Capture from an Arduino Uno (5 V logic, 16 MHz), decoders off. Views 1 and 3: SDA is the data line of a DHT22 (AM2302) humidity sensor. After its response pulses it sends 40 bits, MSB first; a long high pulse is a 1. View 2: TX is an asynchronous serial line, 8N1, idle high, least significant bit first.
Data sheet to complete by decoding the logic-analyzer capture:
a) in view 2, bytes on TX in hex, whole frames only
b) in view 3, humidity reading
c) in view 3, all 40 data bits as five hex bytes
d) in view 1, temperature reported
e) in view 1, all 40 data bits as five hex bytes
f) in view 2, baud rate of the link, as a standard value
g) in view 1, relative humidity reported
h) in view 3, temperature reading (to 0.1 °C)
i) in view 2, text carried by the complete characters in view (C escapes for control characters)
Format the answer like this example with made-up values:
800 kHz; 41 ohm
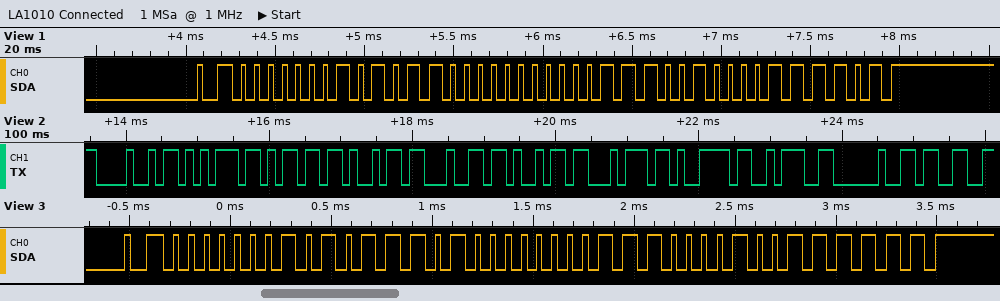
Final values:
48 75 6D 69 64 69 74 79 3A 20 33; 34.9 %; 01 5D 00 E1 3F; 22.8 °C; 01 58 00 E4 3D; 9600 baud; 34.4 %; 22.5 °C; "Humidity: 3"
